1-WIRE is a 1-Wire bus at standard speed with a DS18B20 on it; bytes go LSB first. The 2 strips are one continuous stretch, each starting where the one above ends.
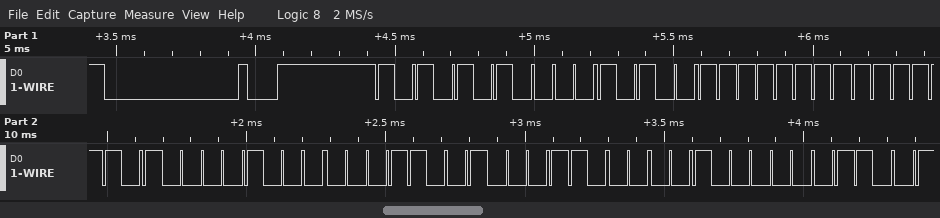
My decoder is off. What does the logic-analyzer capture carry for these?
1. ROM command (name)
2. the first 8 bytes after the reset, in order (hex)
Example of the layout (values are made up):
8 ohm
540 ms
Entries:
Match ROM
55 28 FF BF 10 98 18 04
